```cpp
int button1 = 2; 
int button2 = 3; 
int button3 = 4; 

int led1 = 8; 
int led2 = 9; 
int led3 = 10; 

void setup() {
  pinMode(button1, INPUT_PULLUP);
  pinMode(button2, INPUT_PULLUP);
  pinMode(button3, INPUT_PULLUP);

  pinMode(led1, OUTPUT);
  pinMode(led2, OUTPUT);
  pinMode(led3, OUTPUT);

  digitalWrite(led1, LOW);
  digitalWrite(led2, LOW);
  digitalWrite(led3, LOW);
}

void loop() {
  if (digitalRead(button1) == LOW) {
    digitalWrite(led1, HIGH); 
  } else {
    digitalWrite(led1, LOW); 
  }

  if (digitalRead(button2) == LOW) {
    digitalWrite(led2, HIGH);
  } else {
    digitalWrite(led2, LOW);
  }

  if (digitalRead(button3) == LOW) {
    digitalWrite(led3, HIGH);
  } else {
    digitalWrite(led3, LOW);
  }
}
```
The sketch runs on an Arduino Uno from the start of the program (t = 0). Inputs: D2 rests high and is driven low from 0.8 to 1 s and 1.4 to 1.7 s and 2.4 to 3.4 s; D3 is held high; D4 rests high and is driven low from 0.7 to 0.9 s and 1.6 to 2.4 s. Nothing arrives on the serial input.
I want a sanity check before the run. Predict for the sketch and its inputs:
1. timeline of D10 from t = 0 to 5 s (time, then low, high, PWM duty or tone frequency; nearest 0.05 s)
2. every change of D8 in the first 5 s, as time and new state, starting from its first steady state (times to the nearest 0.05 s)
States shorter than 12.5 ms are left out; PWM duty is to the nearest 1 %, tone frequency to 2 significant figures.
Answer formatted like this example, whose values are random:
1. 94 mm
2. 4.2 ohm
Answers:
1. 0 s low; 0.7 s high; 0.9 s low; 1.6 s high; 2.4 s low
2. 0 s low; 0.8 s high; 1 s low; 1.4 s high; 1.7 s low; 2.4 s high; 3.4 s low
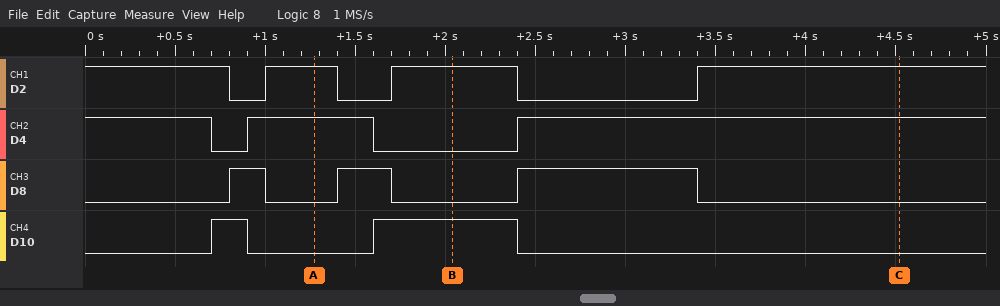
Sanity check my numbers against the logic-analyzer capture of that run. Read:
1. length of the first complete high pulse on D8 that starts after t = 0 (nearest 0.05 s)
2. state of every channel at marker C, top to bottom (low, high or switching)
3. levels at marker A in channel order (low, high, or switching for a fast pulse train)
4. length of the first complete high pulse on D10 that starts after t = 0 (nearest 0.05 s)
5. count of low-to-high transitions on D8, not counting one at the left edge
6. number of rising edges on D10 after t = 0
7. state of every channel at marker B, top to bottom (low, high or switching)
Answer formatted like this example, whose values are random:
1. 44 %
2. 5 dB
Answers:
1. 0.20 s
2. D2 high, D4 high, D8 low, D10 low
3. D2 high, D4 high, D8 low, D10 low
4. 0.20 s
5. 3
6. 2
7. D2 high, D4 low, D8 low, D10 high
